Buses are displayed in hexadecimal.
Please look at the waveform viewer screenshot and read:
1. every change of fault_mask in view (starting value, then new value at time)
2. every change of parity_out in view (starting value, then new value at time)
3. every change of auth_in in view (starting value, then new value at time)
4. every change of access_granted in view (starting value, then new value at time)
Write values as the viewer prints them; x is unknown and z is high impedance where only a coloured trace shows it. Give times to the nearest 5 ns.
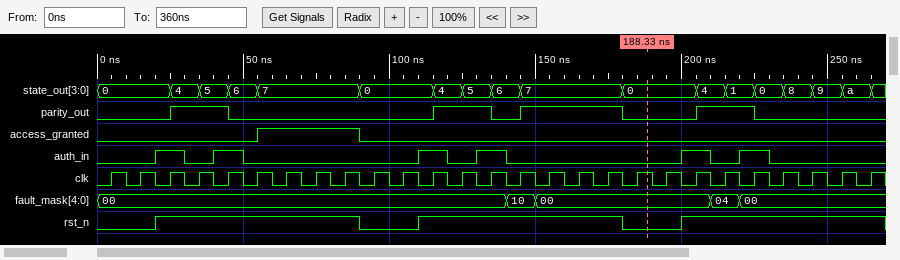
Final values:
00, 10 at 140 ns, 00 at 150 ns, 04 at 210 ns, 00 at 220 ns
0, 1 at 25 ns, 0 at 45 ns, 1 at 115 ns, 0 at 135 ns, 1 at 145 ns, 0 at 180 ns, 1 at 205 ns, 0 at 225 ns
0, 1 at 20 ns, 0 at 30 ns, 1 at 40 ns, 0 at 50 ns, 1 at 110 ns, 0 at 120 ns, 1 at 130 ns, 0 at 140 ns, 1 at 200 ns, 0 at 210 ns, 1 at 220 ns, 0 at 230 ns
0, 1 at 55 ns, 0 at 90 ns
